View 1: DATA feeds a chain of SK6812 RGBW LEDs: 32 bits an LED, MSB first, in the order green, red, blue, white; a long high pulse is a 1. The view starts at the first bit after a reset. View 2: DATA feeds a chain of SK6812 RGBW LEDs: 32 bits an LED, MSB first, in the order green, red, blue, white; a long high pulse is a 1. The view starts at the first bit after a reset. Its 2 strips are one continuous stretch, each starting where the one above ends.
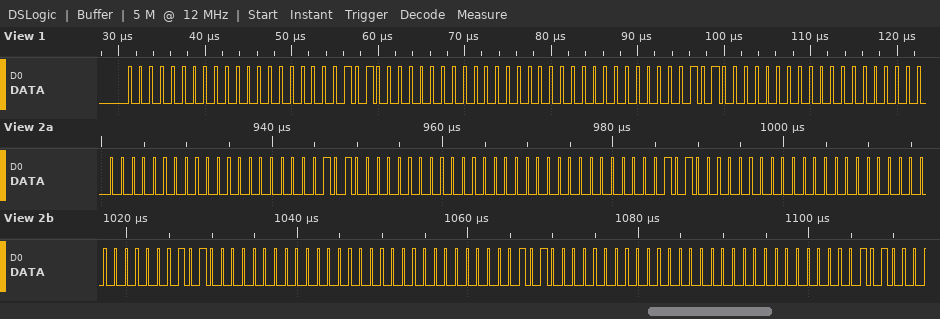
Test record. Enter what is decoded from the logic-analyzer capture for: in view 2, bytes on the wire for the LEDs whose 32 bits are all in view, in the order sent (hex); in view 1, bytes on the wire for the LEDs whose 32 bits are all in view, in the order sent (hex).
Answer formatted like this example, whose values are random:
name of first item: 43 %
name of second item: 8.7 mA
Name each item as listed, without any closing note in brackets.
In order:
in view 2, bytes on the wire for the LEDs whose 32 bits are all in view, in the order sent: 00 00 0A 00 00 00 0A 00 00 00 0A 00 00 00 0A 00
in view 1, bytes on the wire for the LEDs whose 32 bits are all in view, in the order sent: 00 00 0A 00 00 00 0A 00
